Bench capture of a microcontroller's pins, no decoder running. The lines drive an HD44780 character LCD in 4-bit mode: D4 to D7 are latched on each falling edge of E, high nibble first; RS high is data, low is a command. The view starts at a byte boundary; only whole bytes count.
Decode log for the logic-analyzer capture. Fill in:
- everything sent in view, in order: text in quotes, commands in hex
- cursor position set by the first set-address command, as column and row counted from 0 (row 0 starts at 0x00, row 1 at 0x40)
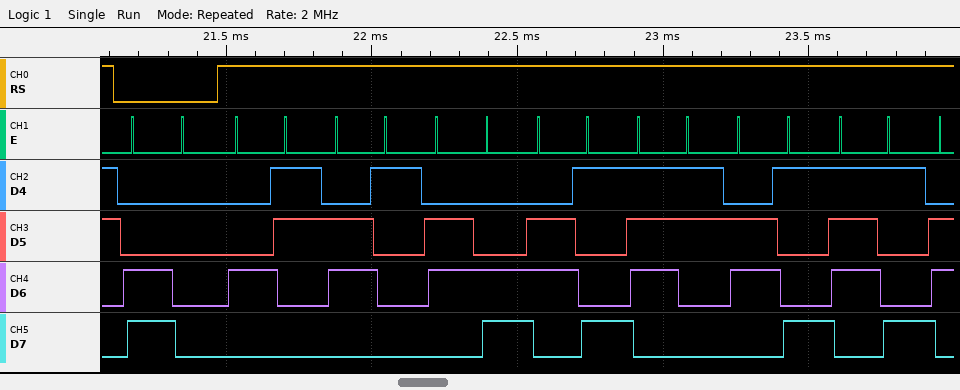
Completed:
0xC0 "Calisiy"
column 0, row 1
